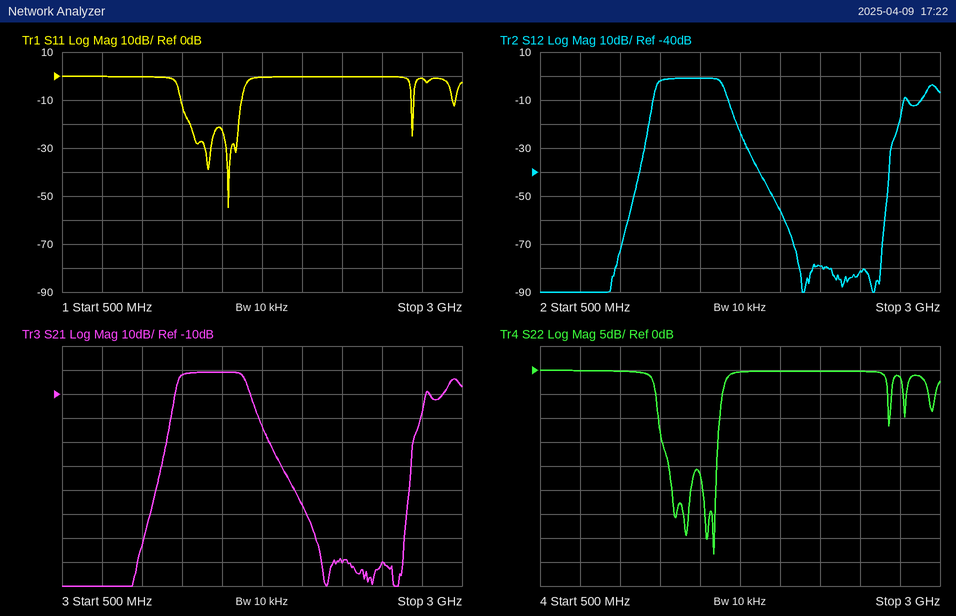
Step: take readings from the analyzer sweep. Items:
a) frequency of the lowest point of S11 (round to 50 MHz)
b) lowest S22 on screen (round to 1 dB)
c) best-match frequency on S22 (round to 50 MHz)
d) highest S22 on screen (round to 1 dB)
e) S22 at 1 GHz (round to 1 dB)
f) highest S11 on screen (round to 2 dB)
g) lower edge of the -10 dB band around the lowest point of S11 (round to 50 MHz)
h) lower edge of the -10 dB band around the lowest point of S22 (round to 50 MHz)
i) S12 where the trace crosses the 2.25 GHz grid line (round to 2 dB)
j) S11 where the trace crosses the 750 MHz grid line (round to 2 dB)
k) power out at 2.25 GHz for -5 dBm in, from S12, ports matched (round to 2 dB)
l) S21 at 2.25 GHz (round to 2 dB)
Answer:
1.55 GHz
-38 dB
1.60 GHz
0 dB
0 dB
0 dB
1.25 GHz
1.25 GHz
-80 dB
0 dB
-84 dBm
-80 dB
